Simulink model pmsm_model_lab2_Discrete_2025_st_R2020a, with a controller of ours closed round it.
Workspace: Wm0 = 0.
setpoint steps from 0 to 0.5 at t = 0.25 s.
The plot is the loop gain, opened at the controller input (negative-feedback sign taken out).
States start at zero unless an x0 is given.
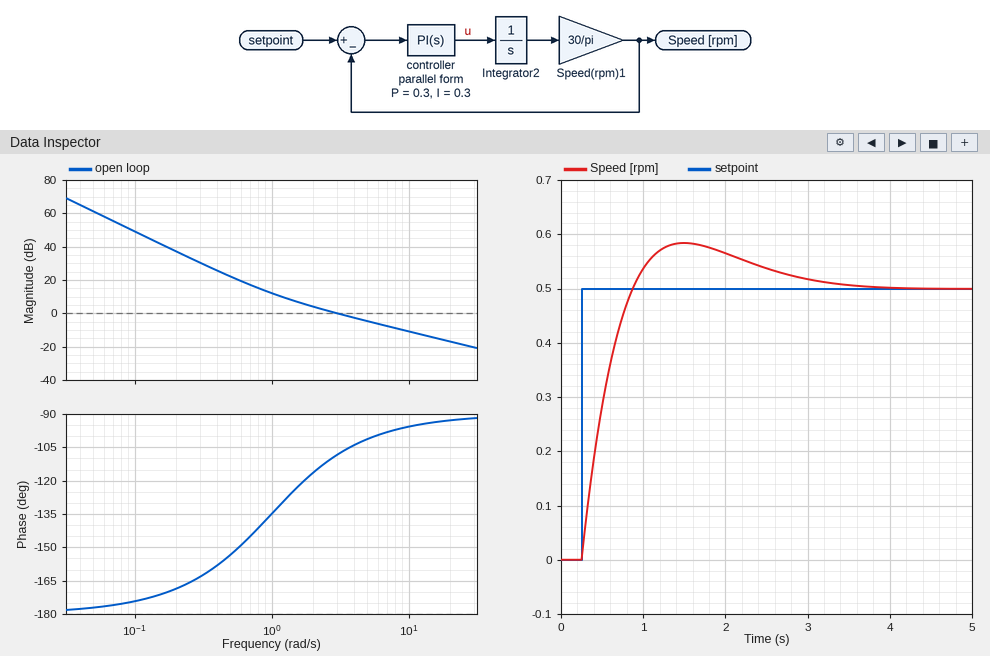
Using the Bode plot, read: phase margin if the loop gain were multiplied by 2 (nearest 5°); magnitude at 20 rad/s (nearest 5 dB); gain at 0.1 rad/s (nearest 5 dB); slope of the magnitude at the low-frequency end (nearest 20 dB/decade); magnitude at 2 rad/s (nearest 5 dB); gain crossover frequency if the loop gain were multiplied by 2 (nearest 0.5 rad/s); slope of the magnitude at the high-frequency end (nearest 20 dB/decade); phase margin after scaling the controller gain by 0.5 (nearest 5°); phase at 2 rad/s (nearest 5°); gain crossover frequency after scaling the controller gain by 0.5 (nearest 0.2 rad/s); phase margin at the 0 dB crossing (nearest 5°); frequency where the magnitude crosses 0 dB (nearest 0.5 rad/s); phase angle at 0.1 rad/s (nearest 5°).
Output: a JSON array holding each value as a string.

["80°", "-15 dB", "50 dB", "-40 dB/decade", "5 dB", "6.0 rad/s", "-20 dB/decade", "60°", "-115°", "1.6 rad/s", "70°", "3.0 rad/s", "-175°"]
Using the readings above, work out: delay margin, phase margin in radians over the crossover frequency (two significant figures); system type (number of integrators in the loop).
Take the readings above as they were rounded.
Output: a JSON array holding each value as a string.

["0.41 s", "2"]
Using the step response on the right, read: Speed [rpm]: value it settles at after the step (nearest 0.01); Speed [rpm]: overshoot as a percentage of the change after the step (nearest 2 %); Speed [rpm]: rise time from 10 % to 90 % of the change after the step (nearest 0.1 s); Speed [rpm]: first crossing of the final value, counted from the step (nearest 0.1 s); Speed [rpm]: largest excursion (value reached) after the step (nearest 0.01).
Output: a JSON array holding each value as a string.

["0.50", "16 %", "0.5 s", "0.6 s", "0.58"]
